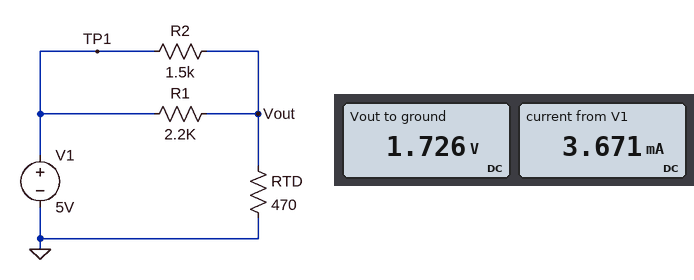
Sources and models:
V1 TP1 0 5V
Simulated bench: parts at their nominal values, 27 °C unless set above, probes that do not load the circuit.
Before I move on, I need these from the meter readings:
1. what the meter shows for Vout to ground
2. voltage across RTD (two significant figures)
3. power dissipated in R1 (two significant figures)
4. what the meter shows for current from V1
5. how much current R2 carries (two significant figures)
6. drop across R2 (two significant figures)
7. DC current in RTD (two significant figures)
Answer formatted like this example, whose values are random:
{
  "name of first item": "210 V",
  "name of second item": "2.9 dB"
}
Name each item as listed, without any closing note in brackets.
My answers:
{
  "what the meter shows for Vout to ground": "1.726 V",
  "voltage across RTD": "1.7 V",
  "power dissipated in R1": "4.9 mW",
  "what the meter shows for current from V1": "3.671 mA",
  "how much current R2 carries": "2.2 mA",
  "drop across R2": "3.3 V",
  "DC current in RTD": "3.7 mA"
}
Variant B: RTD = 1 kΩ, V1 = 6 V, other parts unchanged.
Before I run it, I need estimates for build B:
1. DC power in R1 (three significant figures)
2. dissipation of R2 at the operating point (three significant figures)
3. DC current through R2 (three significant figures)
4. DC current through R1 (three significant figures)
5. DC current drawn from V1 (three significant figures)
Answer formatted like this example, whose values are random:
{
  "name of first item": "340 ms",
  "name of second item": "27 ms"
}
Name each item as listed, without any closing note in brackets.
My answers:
{
  "DC power in R1": "3.64 mW",
  "dissipation of R2 at the operating point": "5.33 mW",
  "DC current through R2": "1.89 mA",
  "DC current through R1": "1.29 mA",
  "DC current drawn from V1": "3.17 mA"
}
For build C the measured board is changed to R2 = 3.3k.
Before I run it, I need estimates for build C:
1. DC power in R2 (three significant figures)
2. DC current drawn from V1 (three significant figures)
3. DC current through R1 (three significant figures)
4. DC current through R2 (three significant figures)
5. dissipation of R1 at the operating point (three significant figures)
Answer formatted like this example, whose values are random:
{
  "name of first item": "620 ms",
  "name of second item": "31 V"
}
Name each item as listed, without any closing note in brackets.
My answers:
{
  "DC power in R2": "4.12 mW",
  "DC current drawn from V1": "2.79 mA",
  "DC current through R1": "1.68 mA",
  "DC current through R2": "1.12 mA",
  "dissipation of R1 at the operating point": "6.18 mW"
}
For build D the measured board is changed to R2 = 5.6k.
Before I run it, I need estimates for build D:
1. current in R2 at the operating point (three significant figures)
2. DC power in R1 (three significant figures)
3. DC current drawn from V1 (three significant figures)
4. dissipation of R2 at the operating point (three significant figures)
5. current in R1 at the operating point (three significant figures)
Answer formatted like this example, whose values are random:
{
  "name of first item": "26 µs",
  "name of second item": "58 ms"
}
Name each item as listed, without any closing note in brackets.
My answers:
{
  "current in R2 at the operating point": "688 µA",
  "DC power in R1": "6.75 mW",
  "DC current drawn from V1": "2.44 mA",
  "dissipation of R2 at the operating point": "2.65 mW",
  "current in R1 at the operating point": "1.75 mA"
}
